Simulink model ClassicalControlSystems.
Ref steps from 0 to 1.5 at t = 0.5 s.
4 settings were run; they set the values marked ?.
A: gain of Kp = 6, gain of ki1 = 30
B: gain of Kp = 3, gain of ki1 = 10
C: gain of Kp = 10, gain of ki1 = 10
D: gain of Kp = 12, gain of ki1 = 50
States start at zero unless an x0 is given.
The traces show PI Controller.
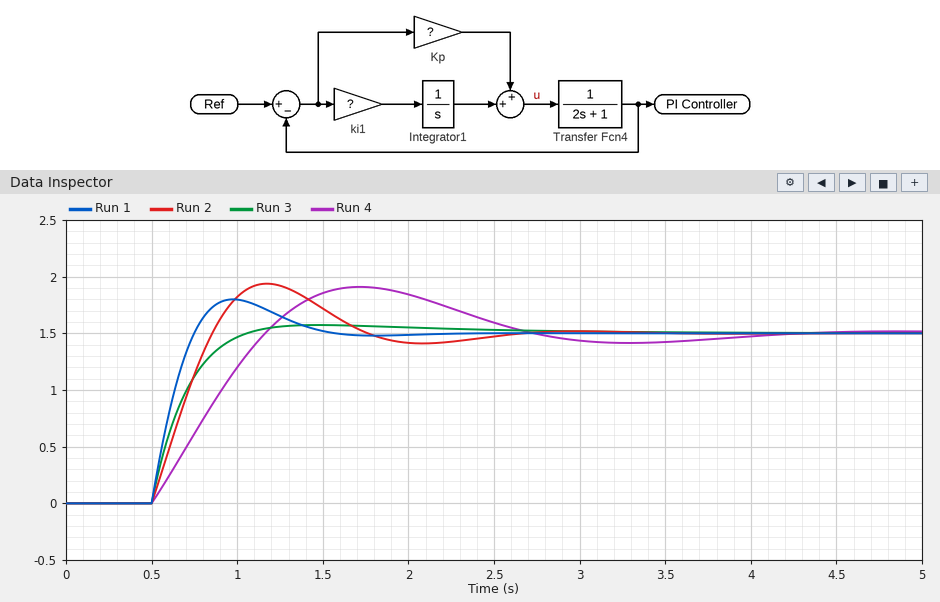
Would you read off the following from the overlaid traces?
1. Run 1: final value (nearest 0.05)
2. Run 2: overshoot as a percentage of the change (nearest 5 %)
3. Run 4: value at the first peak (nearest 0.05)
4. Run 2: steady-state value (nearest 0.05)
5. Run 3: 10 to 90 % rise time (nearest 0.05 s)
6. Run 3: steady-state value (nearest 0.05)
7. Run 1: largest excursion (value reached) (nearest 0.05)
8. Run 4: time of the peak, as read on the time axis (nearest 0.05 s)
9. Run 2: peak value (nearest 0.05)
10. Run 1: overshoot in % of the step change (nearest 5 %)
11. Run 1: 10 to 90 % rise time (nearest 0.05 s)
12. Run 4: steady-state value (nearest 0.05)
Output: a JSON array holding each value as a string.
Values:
["1.50", "30 %", "1.90", "1.50", "0.35 s", "1.50", "1.80", "1.70 s", "1.95", "20 %", "0.20 s", "1.50"]
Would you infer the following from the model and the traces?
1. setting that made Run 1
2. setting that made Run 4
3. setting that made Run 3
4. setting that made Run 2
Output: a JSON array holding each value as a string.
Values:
["D", "B", "C", "A"]
